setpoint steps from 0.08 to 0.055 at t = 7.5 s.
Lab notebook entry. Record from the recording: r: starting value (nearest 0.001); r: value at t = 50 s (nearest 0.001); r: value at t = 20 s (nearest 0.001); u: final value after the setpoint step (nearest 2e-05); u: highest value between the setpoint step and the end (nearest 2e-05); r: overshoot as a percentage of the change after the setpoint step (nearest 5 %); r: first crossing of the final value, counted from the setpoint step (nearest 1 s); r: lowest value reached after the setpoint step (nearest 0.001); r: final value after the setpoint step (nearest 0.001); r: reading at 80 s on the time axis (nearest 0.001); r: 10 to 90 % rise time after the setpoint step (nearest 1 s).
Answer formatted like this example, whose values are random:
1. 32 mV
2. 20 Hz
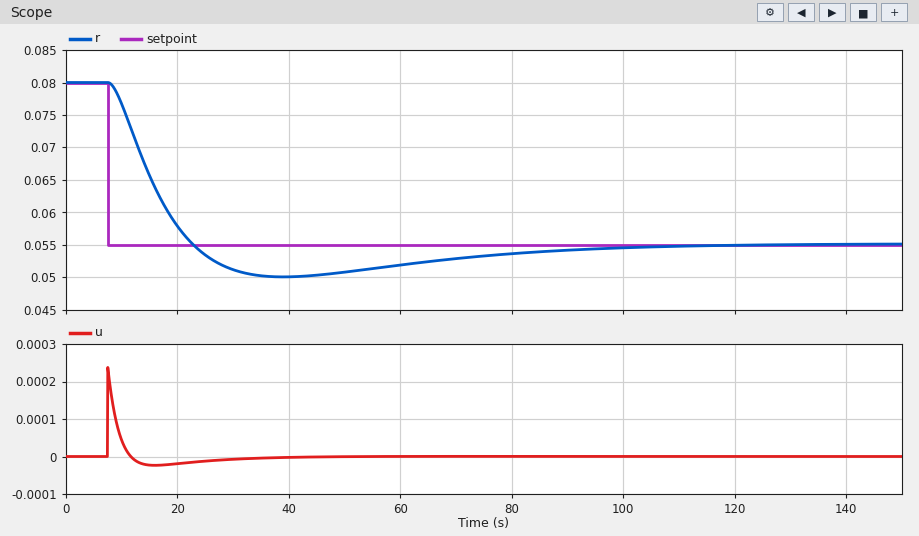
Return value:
1. 0.080
2. 0.051
3. 0.058
4. 0.00000
5. 0.00024
6. 20 %
7. 15 s
8. 0.050
9. 0.055
10. 0.054
11. 11 s
